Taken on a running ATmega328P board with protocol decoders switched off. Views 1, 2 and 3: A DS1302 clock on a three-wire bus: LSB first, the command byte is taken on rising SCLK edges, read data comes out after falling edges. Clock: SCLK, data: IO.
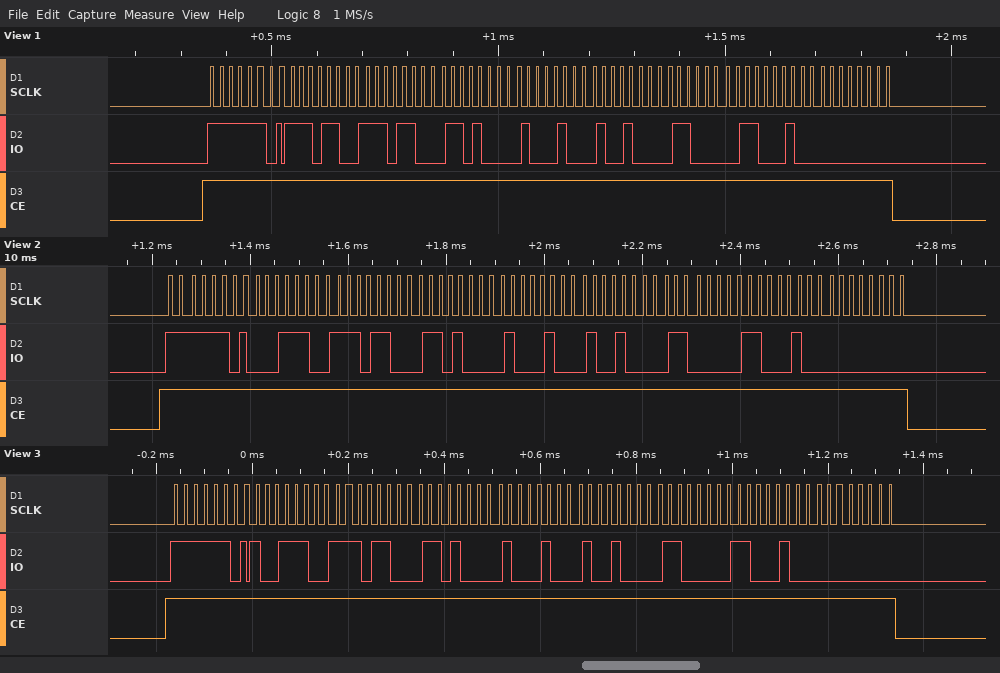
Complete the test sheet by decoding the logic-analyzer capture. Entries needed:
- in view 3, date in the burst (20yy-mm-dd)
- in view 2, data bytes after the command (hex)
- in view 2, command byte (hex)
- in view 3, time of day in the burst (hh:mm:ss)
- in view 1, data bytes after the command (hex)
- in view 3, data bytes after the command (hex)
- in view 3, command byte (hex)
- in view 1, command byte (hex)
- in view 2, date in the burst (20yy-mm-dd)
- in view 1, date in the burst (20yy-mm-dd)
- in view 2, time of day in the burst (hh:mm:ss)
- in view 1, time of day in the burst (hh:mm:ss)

2023-12-22
38 37 16 22 12 06 23 00
0xBF
16:37:39
37 37 16 22 12 06 23 00
39 37 16 22 12 06 23 00
0xBF
0xBF
2023-12-22
2023-12-22
16:37:38
16:37:37
